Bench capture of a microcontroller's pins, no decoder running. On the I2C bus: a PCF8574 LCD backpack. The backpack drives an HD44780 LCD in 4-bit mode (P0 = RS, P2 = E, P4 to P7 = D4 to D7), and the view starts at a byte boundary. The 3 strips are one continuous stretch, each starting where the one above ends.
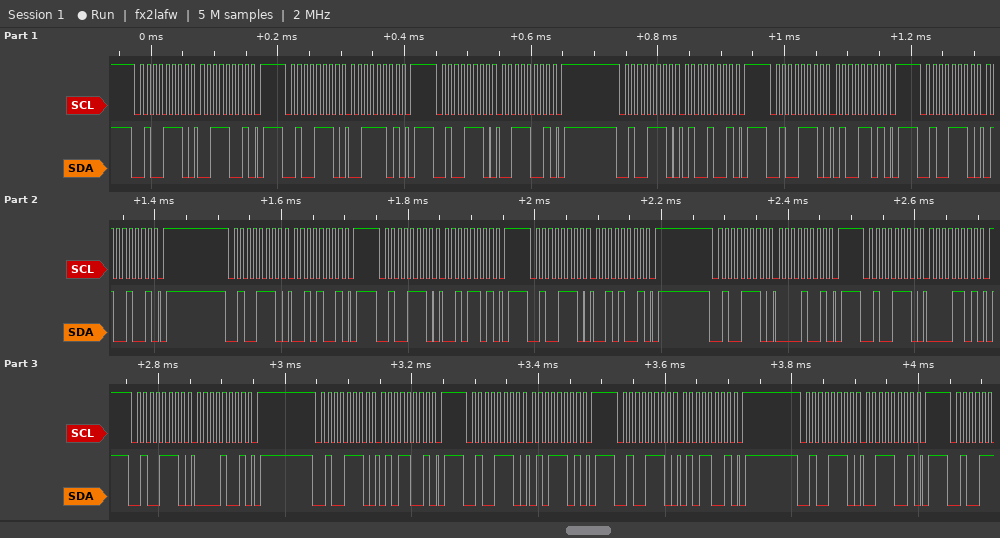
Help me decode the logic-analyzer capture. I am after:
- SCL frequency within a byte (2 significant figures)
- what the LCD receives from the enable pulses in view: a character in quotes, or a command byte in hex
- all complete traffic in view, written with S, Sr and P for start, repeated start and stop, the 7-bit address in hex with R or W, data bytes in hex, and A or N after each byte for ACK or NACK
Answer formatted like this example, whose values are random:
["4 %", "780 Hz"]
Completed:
["100 kHz", "'4' ' '", "S 27W A 39 A P S 27W A 3D A P S 27W A 39 A P S 27W A 49 A P S 27W A 4D A P S 27W A 49 A P S 27W A 29 A P S 27W A 2D A P S 27W A 29 A P S 27W A 09 A P S 27W A 0D A P S 27W A 09 A P S 27W A 59 A P S 27W A 5D A P S 27W A 59 A P S 27W A 39 A P"]
